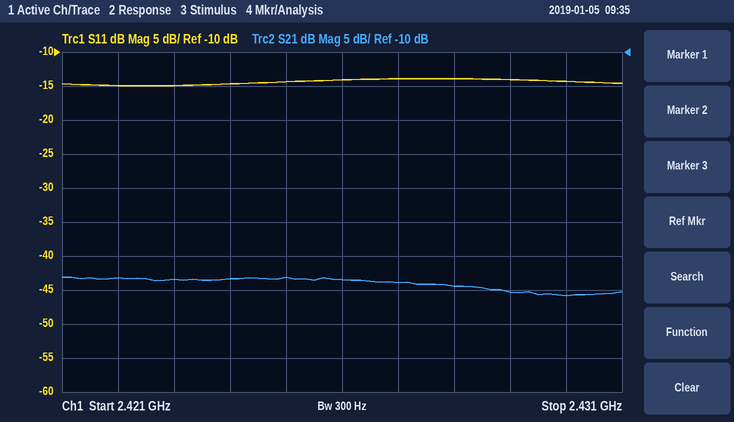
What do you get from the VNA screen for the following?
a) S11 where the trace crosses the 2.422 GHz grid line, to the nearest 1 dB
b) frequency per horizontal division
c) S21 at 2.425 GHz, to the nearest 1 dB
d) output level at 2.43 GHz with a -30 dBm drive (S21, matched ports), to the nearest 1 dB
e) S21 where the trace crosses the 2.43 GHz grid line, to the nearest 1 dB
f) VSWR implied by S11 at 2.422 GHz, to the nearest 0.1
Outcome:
-15 dB
1 MHz
-43 dB
-76 dBm
-46 dB
1.4
